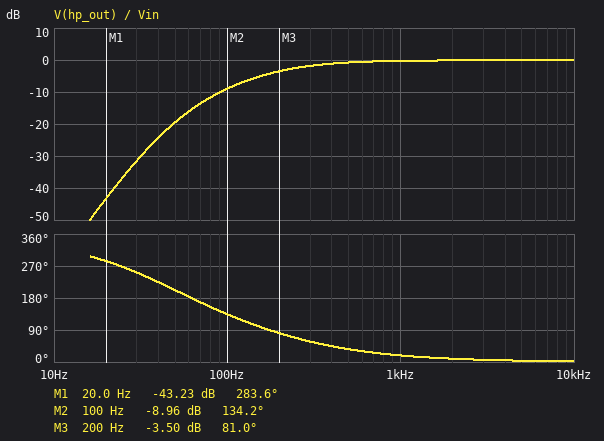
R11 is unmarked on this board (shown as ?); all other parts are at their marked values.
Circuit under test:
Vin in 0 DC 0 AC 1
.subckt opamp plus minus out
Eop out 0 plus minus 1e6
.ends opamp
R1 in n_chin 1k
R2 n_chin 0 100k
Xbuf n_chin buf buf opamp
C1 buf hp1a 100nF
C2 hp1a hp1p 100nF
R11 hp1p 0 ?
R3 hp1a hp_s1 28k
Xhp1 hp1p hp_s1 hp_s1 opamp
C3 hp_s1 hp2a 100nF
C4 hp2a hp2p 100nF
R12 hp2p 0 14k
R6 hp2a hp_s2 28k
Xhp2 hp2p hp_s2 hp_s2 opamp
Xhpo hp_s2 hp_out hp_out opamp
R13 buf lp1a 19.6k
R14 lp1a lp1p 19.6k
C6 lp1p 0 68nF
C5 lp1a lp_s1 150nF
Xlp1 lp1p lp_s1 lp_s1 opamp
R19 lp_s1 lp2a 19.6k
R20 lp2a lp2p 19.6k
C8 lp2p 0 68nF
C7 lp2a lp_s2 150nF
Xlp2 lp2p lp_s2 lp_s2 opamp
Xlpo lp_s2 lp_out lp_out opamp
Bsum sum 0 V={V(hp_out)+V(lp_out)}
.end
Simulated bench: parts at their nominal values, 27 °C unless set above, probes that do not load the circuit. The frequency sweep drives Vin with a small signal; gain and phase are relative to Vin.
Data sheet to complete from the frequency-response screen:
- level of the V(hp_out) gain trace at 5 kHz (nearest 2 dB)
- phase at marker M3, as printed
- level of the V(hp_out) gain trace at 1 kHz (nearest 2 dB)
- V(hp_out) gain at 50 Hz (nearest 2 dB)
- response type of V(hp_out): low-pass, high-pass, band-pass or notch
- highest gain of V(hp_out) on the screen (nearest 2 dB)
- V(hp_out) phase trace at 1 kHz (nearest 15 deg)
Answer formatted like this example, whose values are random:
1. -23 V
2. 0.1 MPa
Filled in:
1. 0 dB
2. 81.0 deg
3. 0 dB
4. -20 dB
5. high-pass
6. 0 dB
7. 15 deg
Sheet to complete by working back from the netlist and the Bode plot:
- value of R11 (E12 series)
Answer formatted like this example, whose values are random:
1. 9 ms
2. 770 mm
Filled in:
1. 33 kΩ
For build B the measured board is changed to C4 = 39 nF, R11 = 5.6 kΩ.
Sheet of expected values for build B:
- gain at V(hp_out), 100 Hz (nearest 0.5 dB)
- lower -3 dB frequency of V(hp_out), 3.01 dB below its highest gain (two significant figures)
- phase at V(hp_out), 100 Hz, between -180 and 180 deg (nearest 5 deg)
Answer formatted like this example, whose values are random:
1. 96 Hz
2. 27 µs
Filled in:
1. -27.5 dB
2. 710 Hz
3. -165 deg
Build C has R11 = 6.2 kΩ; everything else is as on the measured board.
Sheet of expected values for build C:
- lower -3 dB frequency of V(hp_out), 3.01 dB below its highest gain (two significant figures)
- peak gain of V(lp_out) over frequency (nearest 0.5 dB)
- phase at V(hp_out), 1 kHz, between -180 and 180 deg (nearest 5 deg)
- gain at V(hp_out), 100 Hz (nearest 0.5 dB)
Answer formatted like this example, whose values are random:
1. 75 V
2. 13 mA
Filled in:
1. 550 Hz
2. 0 dB
3. 40 deg
4. -21.5 dB
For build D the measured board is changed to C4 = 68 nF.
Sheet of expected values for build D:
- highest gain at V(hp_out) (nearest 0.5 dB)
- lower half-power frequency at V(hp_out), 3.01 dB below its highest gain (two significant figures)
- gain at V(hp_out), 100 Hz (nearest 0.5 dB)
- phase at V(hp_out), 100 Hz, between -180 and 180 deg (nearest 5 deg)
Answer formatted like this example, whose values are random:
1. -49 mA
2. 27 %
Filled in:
1. 0 dB
2. 260 Hz
3. -10.5 dB
4. 140 deg
